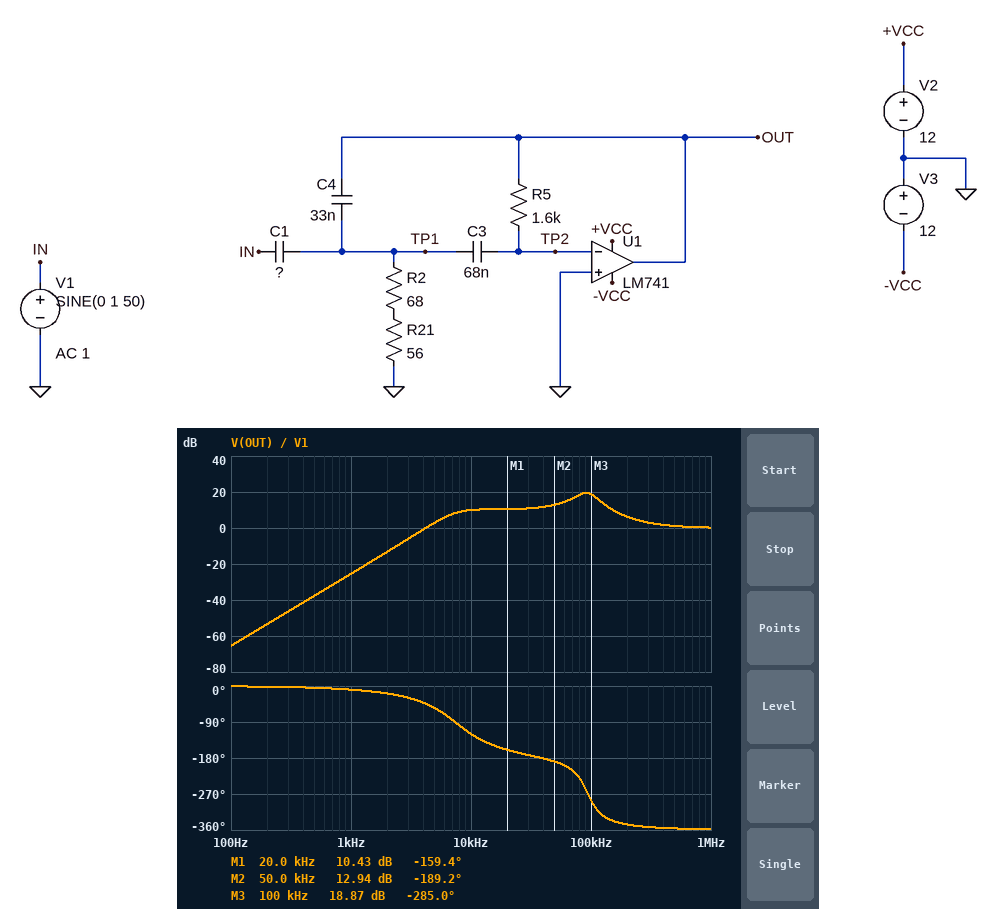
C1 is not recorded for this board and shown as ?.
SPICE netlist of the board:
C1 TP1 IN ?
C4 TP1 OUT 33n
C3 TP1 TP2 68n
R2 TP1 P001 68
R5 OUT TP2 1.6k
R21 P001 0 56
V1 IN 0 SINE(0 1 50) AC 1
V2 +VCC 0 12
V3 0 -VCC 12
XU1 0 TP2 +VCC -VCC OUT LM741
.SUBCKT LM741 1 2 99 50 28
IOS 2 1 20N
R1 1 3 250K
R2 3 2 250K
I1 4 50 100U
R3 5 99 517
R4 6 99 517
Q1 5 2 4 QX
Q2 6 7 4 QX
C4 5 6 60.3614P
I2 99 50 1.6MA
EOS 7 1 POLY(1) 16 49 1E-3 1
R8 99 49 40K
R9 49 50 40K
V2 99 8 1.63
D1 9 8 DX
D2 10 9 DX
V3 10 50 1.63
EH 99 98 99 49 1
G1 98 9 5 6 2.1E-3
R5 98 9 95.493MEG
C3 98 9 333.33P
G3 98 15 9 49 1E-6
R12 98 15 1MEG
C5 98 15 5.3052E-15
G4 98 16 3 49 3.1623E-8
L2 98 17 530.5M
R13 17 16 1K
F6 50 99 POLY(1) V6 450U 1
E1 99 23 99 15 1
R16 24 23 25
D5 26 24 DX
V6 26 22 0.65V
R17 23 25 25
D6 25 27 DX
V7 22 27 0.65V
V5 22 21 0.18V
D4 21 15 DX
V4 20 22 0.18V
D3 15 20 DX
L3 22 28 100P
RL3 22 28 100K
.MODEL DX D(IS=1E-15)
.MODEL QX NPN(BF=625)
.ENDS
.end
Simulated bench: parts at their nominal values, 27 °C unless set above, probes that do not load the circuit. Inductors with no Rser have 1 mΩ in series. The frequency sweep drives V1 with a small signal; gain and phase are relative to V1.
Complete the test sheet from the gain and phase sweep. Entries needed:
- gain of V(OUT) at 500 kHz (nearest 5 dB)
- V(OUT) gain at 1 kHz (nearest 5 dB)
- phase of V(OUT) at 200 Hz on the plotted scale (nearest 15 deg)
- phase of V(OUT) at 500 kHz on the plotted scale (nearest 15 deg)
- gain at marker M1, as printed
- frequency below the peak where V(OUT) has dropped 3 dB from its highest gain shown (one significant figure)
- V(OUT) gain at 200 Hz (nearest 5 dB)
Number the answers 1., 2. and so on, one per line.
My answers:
1. 0 dB
2. -25 dB
3. 0 deg
4. -360 deg
5. 10.43 dB
6. 70 kHz
7. -55 dB
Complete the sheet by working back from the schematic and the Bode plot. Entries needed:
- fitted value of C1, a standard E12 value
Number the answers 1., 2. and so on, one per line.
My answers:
1. 100 nF
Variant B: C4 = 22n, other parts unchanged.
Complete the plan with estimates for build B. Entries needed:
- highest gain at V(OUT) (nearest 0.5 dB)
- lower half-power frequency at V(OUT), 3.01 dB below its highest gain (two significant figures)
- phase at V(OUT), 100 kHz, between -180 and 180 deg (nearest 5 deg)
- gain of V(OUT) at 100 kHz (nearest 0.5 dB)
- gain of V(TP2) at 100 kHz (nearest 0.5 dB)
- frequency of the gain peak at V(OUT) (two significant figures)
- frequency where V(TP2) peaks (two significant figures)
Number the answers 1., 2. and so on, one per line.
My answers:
1. 20.5 dB
2. 60 kHz
3. 80 deg
4. 19.5 dB
5. 6.5 dB
6. 88 kHz
7. 99 kHz
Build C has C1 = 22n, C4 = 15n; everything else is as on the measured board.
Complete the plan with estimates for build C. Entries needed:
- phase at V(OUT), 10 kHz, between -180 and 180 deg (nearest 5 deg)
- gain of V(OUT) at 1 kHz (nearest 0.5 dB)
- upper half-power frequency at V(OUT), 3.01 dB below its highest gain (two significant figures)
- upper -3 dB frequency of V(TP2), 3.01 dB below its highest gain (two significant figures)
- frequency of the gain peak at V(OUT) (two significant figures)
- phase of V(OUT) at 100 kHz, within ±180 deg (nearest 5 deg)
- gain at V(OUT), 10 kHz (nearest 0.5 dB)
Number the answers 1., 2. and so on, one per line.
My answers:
1. -80 deg
2. -38.5 dB
3. 280 kHz
4. 460 kHz
5. 200 kHz
6. 160 deg
7. 3.5 dB
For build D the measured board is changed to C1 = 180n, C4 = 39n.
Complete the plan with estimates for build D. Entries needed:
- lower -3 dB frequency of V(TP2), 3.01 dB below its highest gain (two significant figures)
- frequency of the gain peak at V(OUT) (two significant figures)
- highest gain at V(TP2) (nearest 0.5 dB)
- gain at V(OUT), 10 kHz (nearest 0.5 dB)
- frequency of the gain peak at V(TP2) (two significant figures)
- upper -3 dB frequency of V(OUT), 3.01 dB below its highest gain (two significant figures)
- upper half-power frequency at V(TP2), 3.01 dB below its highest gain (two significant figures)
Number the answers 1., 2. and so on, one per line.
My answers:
1. 60 kHz
2. 67 kHz
3. 9.5 dB
4. 12.0 dB
5. 71 kHz
6. 80 kHz
7. 90 kHz
